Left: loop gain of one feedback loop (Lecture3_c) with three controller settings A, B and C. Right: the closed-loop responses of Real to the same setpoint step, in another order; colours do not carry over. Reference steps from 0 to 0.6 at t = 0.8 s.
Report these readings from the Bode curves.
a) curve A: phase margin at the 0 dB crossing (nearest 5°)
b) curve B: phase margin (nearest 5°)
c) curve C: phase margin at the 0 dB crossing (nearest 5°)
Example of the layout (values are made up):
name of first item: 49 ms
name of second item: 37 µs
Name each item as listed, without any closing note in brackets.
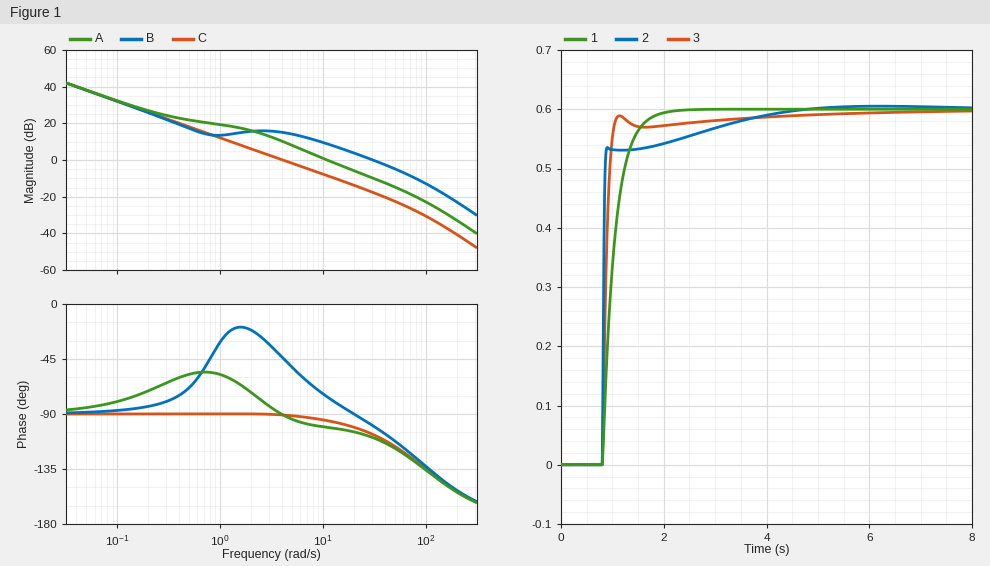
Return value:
curve A: phase margin at the 0 dB crossing: 80°
curve B: phase margin: 80°
curve C: phase margin at the 0 dB crossing: 90°
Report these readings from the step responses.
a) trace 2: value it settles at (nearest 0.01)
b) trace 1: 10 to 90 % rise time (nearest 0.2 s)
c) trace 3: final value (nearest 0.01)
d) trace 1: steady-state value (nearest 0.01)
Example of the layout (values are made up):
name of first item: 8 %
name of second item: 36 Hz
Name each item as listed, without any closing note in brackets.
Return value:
trace 2: value it settles at: 0.60
trace 1: 10 to 90 % rise time: 0.6 s
trace 3: final value: 0.60
trace 1: steady-state value: 0.60
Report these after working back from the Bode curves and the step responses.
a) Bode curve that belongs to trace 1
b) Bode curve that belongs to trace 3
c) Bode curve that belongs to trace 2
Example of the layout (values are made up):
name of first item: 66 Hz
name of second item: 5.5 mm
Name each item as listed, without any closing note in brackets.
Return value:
Bode curve that belongs to trace 1: C
Bode curve that belongs to trace 3: A
Bode curve that belongs to trace 2: B
